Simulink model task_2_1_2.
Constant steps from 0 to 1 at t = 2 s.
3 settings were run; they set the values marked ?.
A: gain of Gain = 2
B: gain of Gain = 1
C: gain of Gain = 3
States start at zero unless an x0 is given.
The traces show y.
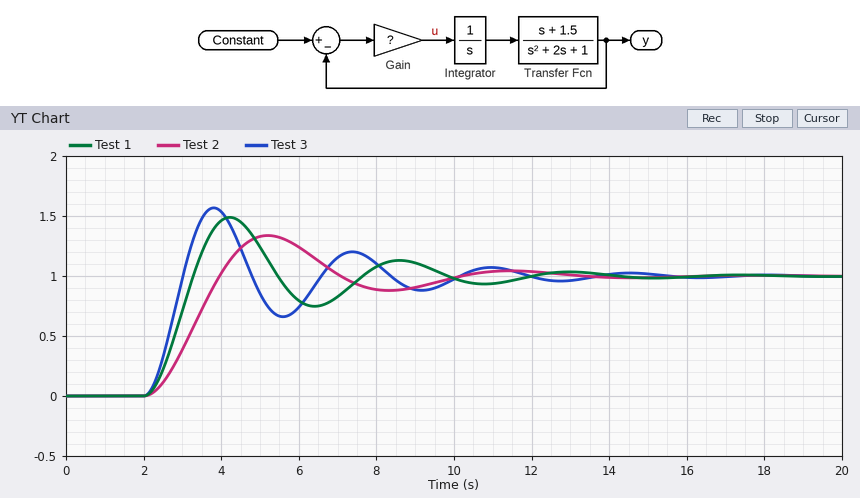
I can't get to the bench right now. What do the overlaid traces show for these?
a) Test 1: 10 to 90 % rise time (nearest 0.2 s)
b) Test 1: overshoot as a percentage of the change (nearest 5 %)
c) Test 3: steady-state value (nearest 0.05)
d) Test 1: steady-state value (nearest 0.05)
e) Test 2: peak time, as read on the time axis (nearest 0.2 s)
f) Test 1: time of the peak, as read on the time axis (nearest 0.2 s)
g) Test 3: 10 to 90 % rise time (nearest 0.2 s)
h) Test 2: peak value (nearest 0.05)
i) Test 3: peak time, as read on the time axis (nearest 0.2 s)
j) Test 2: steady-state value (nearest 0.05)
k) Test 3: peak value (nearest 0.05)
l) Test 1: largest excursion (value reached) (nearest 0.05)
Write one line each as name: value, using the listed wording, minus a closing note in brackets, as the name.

Test 1: 10 to 90 % rise time: 0.8 s
Test 1: overshoot as a percentage of the change: 50 %
Test 3: steady-state value: 1.00
Test 1: steady-state value: 1.00
Test 2: peak time, as read on the time axis: 5.2 s
Test 1: time of the peak, as read on the time axis: 4.2 s
Test 3: 10 to 90 % rise time: 0.6 s
Test 2: peak value: 1.35
Test 3: peak time, as read on the time axis: 3.8 s
Test 2: steady-state value: 1.00
Test 3: peak value: 1.55
Test 1: largest excursion (value reached): 1.50
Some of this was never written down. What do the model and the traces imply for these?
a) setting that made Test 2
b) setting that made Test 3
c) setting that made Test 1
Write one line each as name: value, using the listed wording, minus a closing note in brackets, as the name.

setting that made Test 2: B
setting that made Test 3: C
setting that made Test 1: A
